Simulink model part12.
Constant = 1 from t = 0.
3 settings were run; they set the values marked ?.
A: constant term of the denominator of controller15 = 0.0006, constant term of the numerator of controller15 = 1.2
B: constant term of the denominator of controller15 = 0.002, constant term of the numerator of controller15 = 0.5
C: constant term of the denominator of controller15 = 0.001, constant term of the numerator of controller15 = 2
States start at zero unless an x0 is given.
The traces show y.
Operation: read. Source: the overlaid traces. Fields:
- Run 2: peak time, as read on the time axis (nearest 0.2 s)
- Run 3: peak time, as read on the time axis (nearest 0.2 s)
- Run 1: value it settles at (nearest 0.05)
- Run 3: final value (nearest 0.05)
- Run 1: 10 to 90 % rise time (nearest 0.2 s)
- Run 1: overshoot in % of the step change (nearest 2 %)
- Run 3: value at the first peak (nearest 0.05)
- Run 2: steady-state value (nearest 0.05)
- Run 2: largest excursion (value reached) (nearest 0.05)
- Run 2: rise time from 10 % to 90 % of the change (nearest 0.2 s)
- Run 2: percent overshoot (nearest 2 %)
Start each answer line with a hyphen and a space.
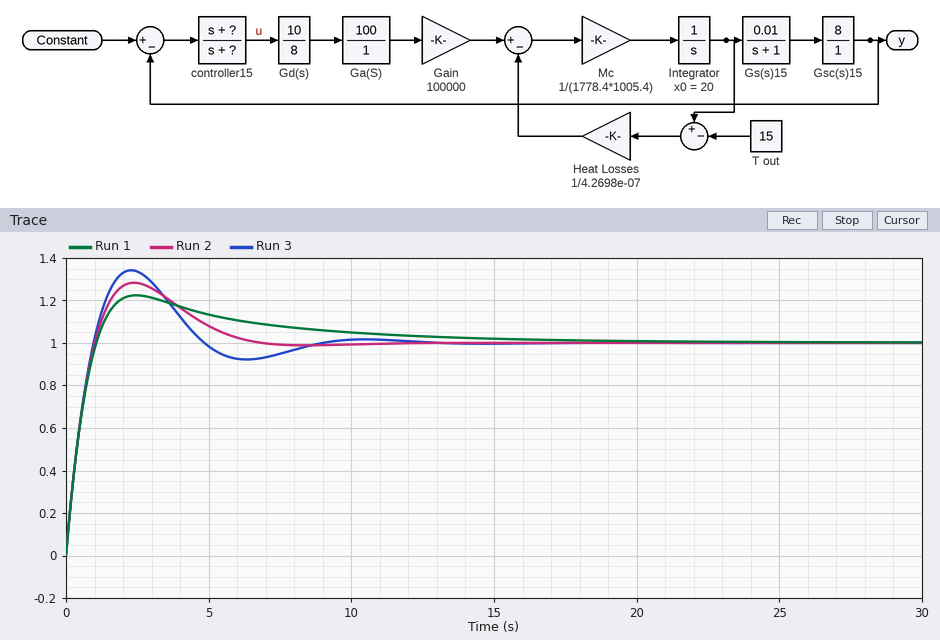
- 2.4 s
- 2.2 s
- 1.00
- 1.00
- 0.8 s
- 22 %
- 1.35
- 1.00
- 1.30
- 0.8 s
- 28 %
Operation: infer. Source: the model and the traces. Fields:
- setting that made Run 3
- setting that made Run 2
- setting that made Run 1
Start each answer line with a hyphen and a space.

- C
- A
- B
